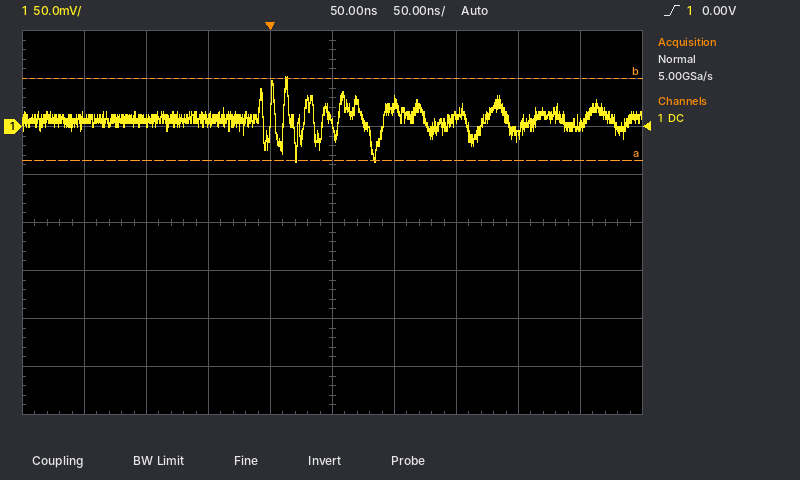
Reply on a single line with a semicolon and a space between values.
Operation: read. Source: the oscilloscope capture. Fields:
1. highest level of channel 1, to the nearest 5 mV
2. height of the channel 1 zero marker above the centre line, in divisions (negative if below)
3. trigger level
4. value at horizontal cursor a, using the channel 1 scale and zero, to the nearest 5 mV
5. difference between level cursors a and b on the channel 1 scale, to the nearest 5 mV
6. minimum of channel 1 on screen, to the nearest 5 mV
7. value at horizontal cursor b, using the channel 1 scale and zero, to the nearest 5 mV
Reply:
50 mV; +2.0 div; 0.00 V; -35 mV; 85 mV; -35 mV; 50 mV
